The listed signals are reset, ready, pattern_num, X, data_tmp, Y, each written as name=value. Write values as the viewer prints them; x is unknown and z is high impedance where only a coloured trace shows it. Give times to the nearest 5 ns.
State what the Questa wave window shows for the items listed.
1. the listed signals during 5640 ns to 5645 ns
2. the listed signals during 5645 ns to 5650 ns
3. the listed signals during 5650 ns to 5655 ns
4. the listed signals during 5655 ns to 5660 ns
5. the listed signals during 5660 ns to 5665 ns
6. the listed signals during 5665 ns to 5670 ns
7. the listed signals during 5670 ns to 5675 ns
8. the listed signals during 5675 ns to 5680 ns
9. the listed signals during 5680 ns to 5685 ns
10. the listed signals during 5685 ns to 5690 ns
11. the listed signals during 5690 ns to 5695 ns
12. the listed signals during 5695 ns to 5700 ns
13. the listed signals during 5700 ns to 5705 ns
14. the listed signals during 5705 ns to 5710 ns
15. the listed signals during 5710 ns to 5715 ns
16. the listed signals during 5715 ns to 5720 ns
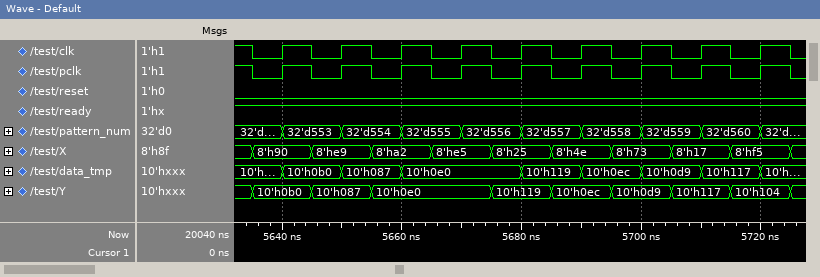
reset=0, ready=1, pattern_num=32'd553, X=8'h90, data_tmp=10'h0b0, Y=10'h0b0
reset=0, ready=1, pattern_num=32'd553, X=8'he9, data_tmp=10'h0b0, Y=10'h087
reset=0, ready=1, pattern_num=32'd554, X=8'he9, data_tmp=10'h087, Y=10'h087
reset=0, ready=1, pattern_num=32'd554, X=8'ha2, data_tmp=10'h087, Y=10'h0e0
reset=0, ready=1, pattern_num=32'd555, X=8'ha2, data_tmp=10'h0e0, Y=10'h0e0
reset=0, ready=1, pattern_num=32'd555, X=8'he5, data_tmp=10'h0e0, Y=10'h0e0
reset=0, ready=1, pattern_num=32'd556, X=8'he5, data_tmp=10'h0e0, Y=10'h0e0
reset=0, ready=1, pattern_num=32'd556, X=8'h25, data_tmp=10'h0e0, Y=10'h119
reset=0, ready=1, pattern_num=32'd557, X=8'h25, data_tmp=10'h119, Y=10'h119
reset=0, ready=1, pattern_num=32'd557, X=8'h4e, data_tmp=10'h119, Y=10'h0ec
reset=0, ready=1, pattern_num=32'd558, X=8'h4e, data_tmp=10'h0ec, Y=10'h0ec
reset=0, ready=1, pattern_num=32'd558, X=8'h73, data_tmp=10'h0ec, Y=10'h0d9
reset=0, ready=1, pattern_num=32'd559, X=8'h73, data_tmp=10'h0d9, Y=10'h0d9
reset=0, ready=1, pattern_num=32'd559, X=8'h17, data_tmp=10'h0d9, Y=10'h117
reset=0, ready=1, pattern_num=32'd560, X=8'h17, data_tmp=10'h117, Y=10'h117
reset=0, ready=1, pattern_num=32'd560, X=8'hf5, data_tmp=10'h117, Y=10'h104
